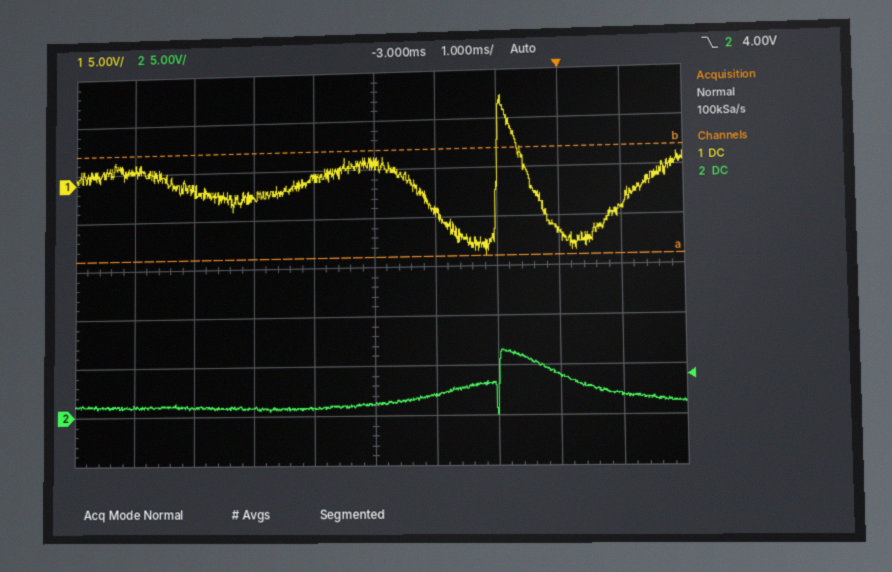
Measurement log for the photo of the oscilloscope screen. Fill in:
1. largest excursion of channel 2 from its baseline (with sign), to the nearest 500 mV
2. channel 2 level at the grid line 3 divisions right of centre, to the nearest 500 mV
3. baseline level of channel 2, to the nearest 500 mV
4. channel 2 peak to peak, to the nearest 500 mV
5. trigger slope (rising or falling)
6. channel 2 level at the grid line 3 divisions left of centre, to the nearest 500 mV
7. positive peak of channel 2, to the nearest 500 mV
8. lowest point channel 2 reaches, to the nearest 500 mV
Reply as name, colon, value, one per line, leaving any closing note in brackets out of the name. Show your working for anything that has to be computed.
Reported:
largest excursion of channel 2 from its baseline (with sign), to the nearest 500 mV: 6.5 V − (1.0 V) = +5.5 V
channel 2 level at the grid line 3 divisions right of centre, to the nearest 500 mV: 4.0 V
baseline level of channel 2, to the nearest 500 mV: 1.0 V
channel 2 peak to peak, to the nearest 500 mV: 6.5 V − (0.0 V) = 6.5 V
trigger slope: falling
channel 2 level at the grid line 3 divisions left of centre, to the nearest 500 mV: 1.0 V
positive peak of channel 2, to the nearest 500 mV: 6.5 V
lowest point channel 2 reaches, to the nearest 500 mV: 0.0 V
